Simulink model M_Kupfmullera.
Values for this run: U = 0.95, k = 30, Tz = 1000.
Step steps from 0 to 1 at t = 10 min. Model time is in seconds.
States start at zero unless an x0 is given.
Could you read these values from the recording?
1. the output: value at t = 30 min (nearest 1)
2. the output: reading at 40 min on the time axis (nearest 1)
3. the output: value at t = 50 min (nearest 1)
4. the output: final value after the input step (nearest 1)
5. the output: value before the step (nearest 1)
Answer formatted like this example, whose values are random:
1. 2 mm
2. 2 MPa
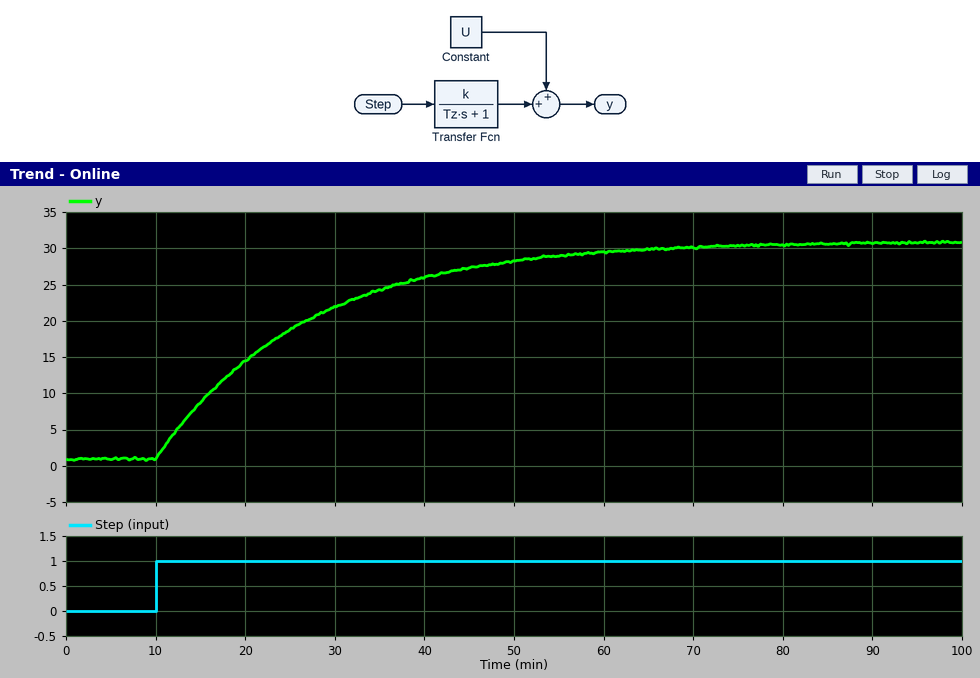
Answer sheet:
1. 22
2. 26
3. 28
4. 31
5. 1
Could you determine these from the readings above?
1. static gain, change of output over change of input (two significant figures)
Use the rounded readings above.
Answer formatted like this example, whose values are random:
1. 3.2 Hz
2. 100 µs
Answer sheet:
1. 30
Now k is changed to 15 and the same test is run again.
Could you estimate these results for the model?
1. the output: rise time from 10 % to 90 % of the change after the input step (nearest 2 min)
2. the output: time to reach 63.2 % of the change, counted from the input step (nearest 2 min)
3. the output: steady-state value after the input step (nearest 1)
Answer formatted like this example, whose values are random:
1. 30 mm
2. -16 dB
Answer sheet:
1. 36 min
2. 16 min
3. 16
